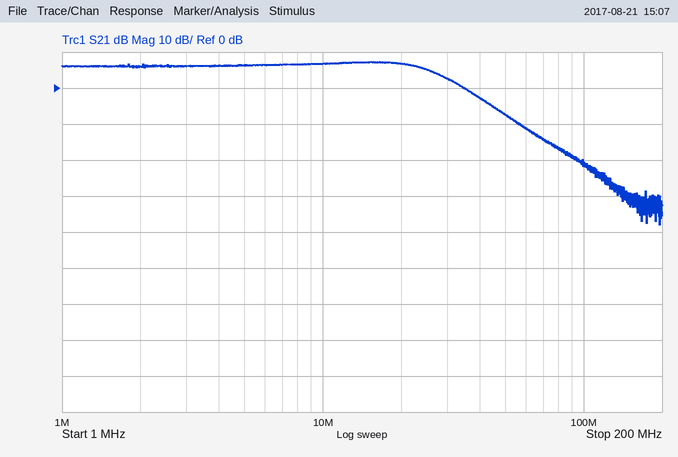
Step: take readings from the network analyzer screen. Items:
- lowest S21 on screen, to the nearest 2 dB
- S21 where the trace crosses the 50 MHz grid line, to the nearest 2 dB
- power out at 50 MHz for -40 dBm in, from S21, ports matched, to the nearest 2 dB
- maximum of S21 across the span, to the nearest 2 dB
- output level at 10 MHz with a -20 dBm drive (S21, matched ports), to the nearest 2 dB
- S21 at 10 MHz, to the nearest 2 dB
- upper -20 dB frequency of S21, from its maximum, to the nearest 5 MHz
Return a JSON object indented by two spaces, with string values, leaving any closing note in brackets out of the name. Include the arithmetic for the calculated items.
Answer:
{
  "lowest S21 on screen, to the nearest 2 dB": "-38 dB",
  "S21 where the trace crosses the 50 MHz grid line, to the nearest 2 dB": "-8 dB",
  "power out at 50 MHz for -40 dBm in, from S21, ports matched, to the nearest 2 dB": "-40 dBm + (-8 dB) = -48 dBm",
  "maximum of S21 across the span, to the nearest 2 dB": "8 dB",
  "output level at 10 MHz with a -20 dBm drive (S21, matched ports), to the nearest 2 dB": "-20 dBm + (6 dB) = -14 dBm",
  "S21 at 10 MHz, to the nearest 2 dB": "6 dB",
  "upper -20 dB frequency of S21, from its maximum, to the nearest 5 MHz": "65 MHz"
}
